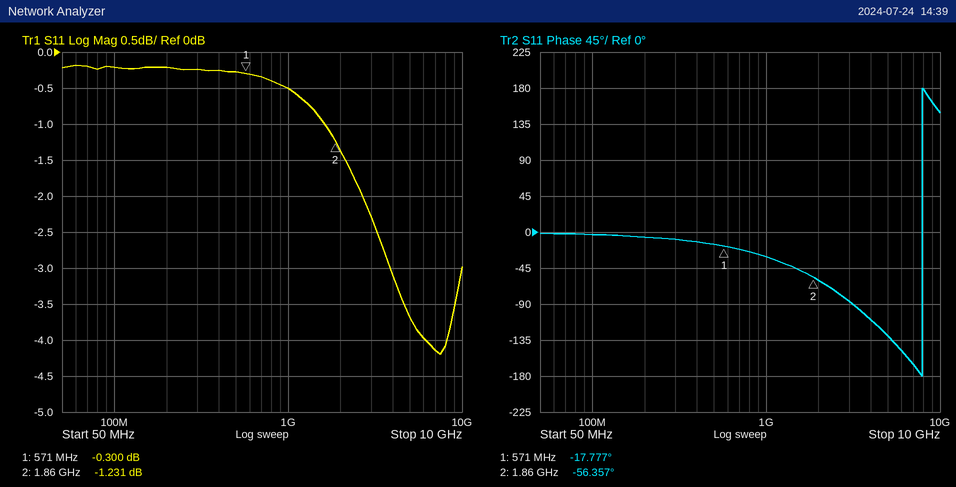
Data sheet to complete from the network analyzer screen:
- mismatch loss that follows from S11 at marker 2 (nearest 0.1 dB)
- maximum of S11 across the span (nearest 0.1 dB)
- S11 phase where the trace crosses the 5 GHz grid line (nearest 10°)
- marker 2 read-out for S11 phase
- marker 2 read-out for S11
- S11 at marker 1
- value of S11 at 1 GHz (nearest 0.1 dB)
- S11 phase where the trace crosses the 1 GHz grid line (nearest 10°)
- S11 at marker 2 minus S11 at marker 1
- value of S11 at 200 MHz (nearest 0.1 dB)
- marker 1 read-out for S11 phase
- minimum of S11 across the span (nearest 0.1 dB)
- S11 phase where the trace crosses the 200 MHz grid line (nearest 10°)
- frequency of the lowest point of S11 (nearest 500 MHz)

6.1 dB
-0.2 dB
-130°
-56.357°
-1.231 dB
-0.300 dB
-0.5 dB
-30°
-0.931 dB
-0.2 dB
-17.777°
-4.2 dB
-10°
7.5 GHz
